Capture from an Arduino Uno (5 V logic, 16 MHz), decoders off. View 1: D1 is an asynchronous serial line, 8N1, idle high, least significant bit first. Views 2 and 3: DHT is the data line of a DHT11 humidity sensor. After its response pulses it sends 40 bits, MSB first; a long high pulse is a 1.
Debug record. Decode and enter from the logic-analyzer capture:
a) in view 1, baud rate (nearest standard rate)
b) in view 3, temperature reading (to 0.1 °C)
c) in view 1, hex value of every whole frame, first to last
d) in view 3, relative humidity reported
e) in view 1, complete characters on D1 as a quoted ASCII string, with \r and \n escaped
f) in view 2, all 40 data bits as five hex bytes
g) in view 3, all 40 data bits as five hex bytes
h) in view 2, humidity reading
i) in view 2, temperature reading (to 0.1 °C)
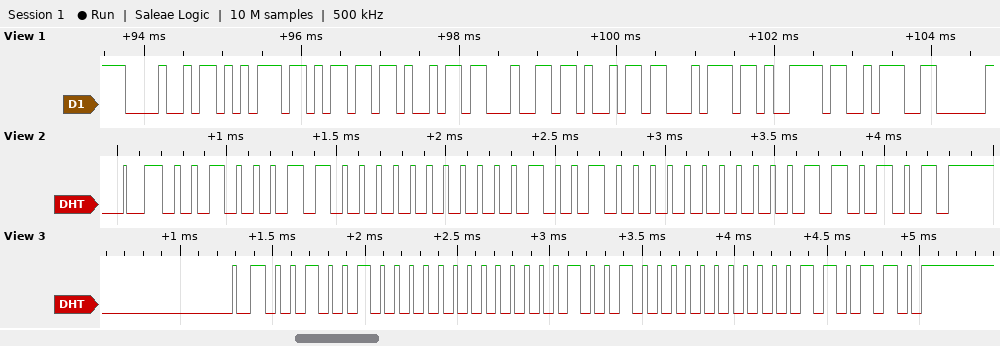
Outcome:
9600 baud
18.0 °C
0x48 0x75 0x6D 0x69 0x64 0x69 0x74 0x79 0x3A
36 %
"Humidity:"
23 00 12 00 35
24 00 12 00 36
35 %
18.0 °C
